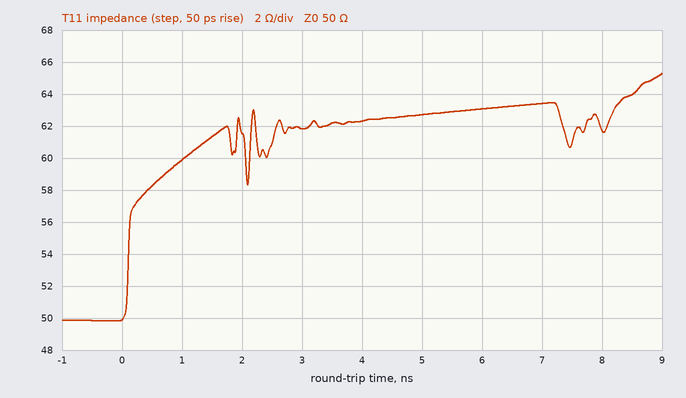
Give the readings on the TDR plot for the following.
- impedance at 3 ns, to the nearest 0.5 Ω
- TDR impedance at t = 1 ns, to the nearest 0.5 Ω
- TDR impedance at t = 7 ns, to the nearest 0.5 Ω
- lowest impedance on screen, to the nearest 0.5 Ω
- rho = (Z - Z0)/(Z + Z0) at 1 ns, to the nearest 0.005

62.0 Ω
60.0 Ω
63.5 Ω
50.0 Ω
+0.090
